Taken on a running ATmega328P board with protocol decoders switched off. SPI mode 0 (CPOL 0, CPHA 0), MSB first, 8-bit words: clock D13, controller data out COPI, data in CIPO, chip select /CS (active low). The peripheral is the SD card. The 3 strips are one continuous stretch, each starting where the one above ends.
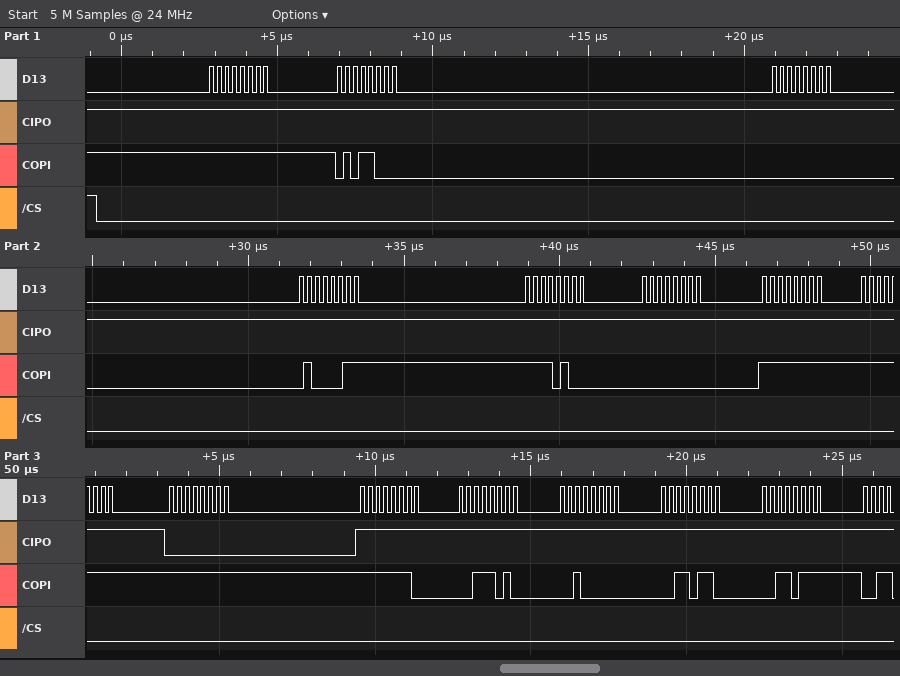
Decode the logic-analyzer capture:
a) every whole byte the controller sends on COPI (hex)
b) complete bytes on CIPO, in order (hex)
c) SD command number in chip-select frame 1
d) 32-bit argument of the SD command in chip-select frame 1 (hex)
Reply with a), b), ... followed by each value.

a) FF 58 00 43 F4 00 FF FF FF FE 3A 20 36 37
b) FF FF FF FF FF FF FF FF 00 FF FF FF FF FF
c) CMD24
d) 0x0043F400
